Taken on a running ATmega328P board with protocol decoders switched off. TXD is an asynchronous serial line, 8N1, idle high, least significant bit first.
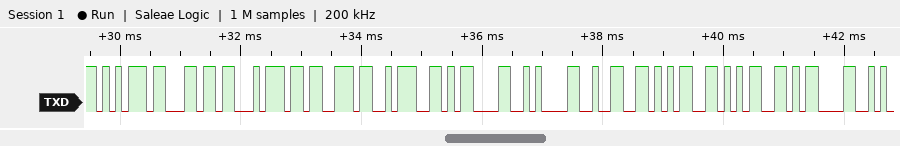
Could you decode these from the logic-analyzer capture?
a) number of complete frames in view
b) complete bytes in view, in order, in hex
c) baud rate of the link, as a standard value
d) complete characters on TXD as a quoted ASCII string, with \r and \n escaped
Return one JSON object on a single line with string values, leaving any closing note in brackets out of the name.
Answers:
{"number of complete frames in view": "11", "complete bytes in view, in order, in hex": "0x75 0x6C 0x74 0x73 0x3A 0x0D 0x0A 0x32 0x35 0x35 0x0D", "baud rate of the link, as a standard value": "9600 baud", "complete characters on TXD as a quoted ASCII string, with \\r and \\n escaped": "\"ults:\\r\\n255\\r\""}
